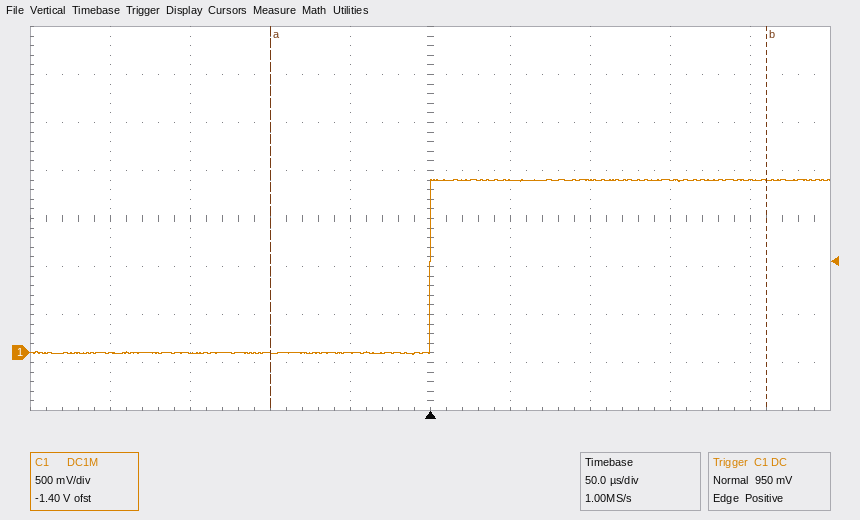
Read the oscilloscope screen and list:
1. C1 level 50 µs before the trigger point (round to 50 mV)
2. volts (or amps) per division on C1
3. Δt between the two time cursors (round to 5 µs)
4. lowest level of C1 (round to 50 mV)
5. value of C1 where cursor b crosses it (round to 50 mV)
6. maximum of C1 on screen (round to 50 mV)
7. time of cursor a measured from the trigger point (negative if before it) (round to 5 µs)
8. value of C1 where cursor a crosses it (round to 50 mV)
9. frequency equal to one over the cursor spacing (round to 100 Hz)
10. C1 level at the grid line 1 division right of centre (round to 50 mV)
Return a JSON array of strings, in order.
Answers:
["0 mV", "500 mV", "310 µs", "0 mV", "1.80 V", "1.80 V", "-100 µs", "0 mV", "3.2 kHz", "1.80 V"]
